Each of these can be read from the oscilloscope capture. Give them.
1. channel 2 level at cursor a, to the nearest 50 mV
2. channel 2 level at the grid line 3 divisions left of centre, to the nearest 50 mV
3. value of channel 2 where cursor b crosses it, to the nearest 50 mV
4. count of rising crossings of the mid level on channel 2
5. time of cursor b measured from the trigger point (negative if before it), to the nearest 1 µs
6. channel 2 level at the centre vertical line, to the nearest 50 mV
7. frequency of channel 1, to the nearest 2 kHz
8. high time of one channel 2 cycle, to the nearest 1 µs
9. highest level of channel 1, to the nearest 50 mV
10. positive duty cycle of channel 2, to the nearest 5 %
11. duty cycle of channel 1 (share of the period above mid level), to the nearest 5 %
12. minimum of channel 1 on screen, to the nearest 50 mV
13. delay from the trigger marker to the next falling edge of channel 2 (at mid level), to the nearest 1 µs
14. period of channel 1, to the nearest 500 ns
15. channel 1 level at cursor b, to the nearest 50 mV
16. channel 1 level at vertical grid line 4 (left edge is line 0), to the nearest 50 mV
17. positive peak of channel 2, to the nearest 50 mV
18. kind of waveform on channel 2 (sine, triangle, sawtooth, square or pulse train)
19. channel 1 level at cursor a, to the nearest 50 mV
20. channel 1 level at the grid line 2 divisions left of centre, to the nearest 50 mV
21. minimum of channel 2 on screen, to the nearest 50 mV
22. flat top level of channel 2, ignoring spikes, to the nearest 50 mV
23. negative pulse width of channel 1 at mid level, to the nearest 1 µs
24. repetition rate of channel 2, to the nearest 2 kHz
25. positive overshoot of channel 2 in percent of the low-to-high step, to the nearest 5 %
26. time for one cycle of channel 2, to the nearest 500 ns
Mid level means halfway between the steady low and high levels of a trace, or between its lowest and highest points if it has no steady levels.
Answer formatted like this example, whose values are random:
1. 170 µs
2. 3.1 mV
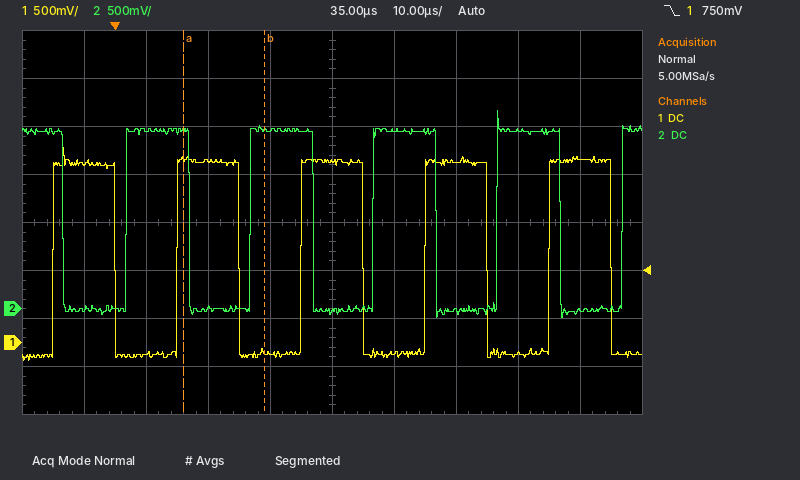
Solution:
1. 1.85 V
2. 1.85 V
3. 1.85 V
4. 5
5. +24 µs
6. -50 mV
7. 50 kHz
8. 10 µs
9. 2.05 V
10. 50 %
11. 50 %
12. -200 mV
13. 12 µs
14. 20.0 µs
15. -100 mV
16. -100 mV
17. 2.05 V
18. square
19. 1.90 V
20. 1.90 V
21. -100 mV
22. 1.85 V
23. 10 µs
24. 50 kHz
25. 10 %
26. 20.0 µs
